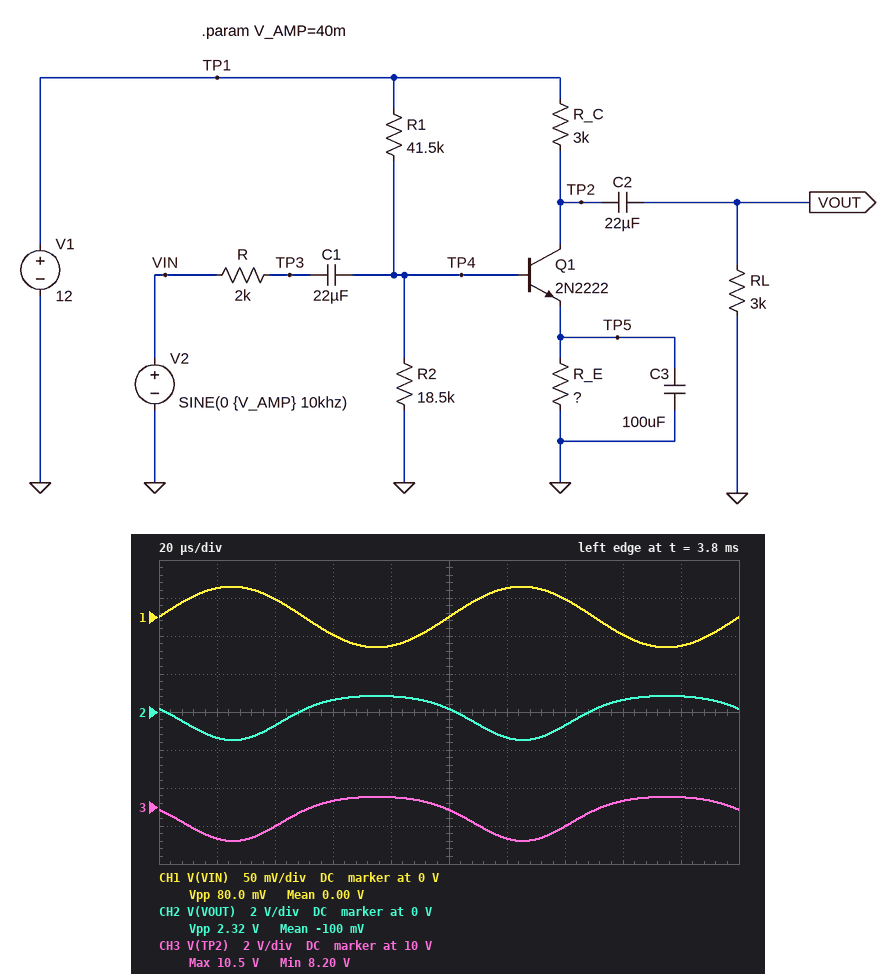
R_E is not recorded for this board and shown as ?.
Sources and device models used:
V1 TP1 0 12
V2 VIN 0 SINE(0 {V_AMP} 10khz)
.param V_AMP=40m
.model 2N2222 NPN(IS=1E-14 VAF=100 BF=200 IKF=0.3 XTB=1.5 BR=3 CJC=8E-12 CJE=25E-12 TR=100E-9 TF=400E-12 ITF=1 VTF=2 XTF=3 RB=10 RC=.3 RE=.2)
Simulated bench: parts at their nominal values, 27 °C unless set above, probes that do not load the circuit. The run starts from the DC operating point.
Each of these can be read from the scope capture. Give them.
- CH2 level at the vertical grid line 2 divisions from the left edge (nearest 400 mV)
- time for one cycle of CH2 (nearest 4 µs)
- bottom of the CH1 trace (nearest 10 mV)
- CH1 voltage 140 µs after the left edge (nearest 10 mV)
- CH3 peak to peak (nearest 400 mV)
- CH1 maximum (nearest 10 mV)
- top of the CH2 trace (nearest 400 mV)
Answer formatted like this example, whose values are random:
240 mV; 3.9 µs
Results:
-800 mV; 100 µs; -40 mV; 20 mV; 2.4 V; 40 mV; 800 mV
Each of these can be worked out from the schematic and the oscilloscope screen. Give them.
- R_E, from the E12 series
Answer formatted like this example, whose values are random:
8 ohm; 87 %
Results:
3.9 kΩ
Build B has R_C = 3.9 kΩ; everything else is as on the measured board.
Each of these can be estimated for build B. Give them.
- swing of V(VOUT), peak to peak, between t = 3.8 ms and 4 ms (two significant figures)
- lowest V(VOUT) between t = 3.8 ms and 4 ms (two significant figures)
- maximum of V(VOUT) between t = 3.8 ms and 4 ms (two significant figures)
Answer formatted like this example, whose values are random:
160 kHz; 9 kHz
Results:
2.6 V; -1.7 V; 950 mV
